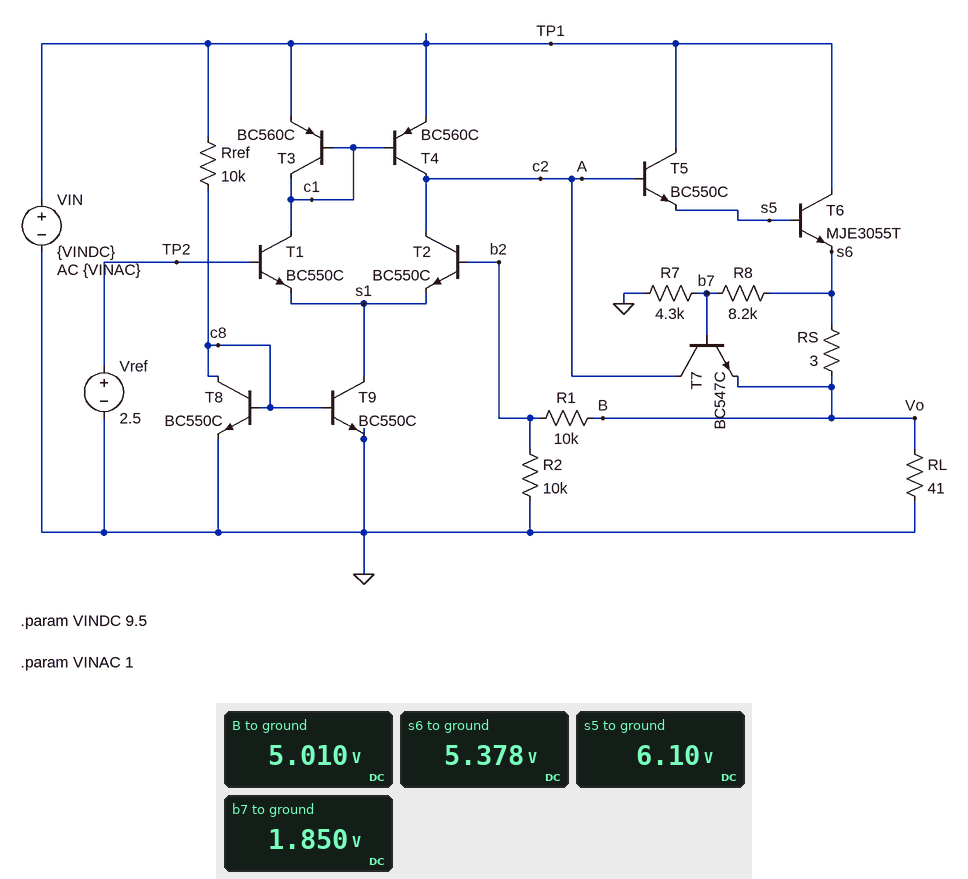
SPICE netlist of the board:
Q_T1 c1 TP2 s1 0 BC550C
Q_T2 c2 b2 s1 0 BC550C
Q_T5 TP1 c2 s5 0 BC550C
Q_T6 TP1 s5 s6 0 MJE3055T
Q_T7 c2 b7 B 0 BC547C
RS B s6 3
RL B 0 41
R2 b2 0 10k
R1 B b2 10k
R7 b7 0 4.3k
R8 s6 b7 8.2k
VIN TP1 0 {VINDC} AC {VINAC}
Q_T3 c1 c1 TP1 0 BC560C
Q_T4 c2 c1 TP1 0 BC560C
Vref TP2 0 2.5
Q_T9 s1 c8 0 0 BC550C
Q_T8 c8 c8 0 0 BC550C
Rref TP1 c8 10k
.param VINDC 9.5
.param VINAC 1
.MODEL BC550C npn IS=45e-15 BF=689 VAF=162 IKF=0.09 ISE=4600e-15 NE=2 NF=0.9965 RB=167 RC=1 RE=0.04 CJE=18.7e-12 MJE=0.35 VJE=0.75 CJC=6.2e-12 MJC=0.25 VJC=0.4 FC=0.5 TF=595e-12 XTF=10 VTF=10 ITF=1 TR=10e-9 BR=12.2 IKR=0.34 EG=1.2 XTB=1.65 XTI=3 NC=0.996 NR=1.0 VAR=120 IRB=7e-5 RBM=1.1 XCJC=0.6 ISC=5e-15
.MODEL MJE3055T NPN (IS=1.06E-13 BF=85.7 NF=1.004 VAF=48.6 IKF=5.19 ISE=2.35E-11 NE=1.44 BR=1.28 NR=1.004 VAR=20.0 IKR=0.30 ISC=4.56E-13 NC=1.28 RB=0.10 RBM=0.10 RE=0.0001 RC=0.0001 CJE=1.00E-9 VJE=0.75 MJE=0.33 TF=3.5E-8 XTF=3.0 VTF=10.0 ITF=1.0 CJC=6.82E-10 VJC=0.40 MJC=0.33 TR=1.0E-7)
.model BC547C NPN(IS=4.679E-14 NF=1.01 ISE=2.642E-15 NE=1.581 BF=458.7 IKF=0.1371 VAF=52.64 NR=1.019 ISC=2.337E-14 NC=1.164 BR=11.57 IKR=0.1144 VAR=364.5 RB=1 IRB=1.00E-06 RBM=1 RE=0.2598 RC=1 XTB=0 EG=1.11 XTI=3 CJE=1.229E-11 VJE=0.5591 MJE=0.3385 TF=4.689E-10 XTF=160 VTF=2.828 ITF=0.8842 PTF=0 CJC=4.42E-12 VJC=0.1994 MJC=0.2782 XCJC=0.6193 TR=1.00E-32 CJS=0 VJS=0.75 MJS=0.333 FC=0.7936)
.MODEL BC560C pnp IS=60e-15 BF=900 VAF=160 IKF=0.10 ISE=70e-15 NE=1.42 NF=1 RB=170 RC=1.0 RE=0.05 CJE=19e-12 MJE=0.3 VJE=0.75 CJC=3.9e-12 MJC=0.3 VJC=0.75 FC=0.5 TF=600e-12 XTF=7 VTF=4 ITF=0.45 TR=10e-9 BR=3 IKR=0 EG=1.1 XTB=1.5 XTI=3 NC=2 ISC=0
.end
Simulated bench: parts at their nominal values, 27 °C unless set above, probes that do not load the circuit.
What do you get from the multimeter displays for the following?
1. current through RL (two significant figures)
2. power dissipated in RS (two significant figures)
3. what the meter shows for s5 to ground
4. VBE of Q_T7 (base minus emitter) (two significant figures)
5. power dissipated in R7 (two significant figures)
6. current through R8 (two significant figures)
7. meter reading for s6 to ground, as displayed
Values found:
120 mA
45 mW
6.10 V
-3.2 V
800 µW
430 µA
5.378 V
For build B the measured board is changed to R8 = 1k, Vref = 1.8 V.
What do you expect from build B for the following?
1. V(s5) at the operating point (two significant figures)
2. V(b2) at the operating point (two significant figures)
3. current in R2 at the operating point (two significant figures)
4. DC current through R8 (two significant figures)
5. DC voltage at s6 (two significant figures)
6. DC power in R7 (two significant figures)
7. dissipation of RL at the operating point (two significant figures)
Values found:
4.6 V
1.8 V
180 µA
730 µA
3.9 V
2.3 mW
320 mW
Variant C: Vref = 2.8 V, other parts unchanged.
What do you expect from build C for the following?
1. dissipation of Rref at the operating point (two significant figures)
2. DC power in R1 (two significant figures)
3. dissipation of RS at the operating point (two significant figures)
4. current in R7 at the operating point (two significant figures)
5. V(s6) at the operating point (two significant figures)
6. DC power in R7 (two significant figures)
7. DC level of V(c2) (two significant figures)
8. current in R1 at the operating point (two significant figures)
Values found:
7.9 mW
790 µW
56 mW
480 µA
6.0 V
1.0 mW
7.4 V
280 µA
